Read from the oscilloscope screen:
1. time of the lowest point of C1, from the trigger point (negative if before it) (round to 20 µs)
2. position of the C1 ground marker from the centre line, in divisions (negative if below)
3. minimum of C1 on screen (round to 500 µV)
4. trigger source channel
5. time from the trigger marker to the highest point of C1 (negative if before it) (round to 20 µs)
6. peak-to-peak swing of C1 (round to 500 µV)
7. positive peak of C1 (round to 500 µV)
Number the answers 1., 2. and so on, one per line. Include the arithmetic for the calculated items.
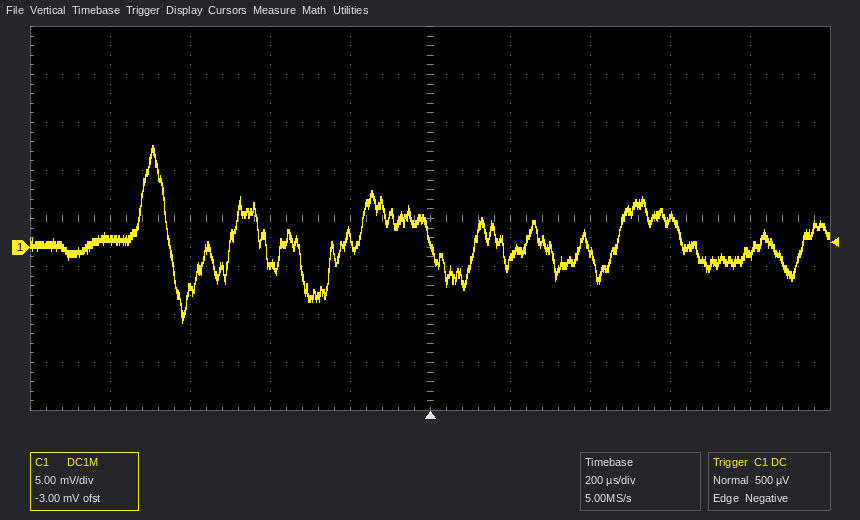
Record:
1. -620 µs
2. -0.6 div
3. -8.0 mV
4. C1
5. -700 µs
6. 10.5 mV − (-8.0 mV) = 18.5 mV
7. 10.5 mV
